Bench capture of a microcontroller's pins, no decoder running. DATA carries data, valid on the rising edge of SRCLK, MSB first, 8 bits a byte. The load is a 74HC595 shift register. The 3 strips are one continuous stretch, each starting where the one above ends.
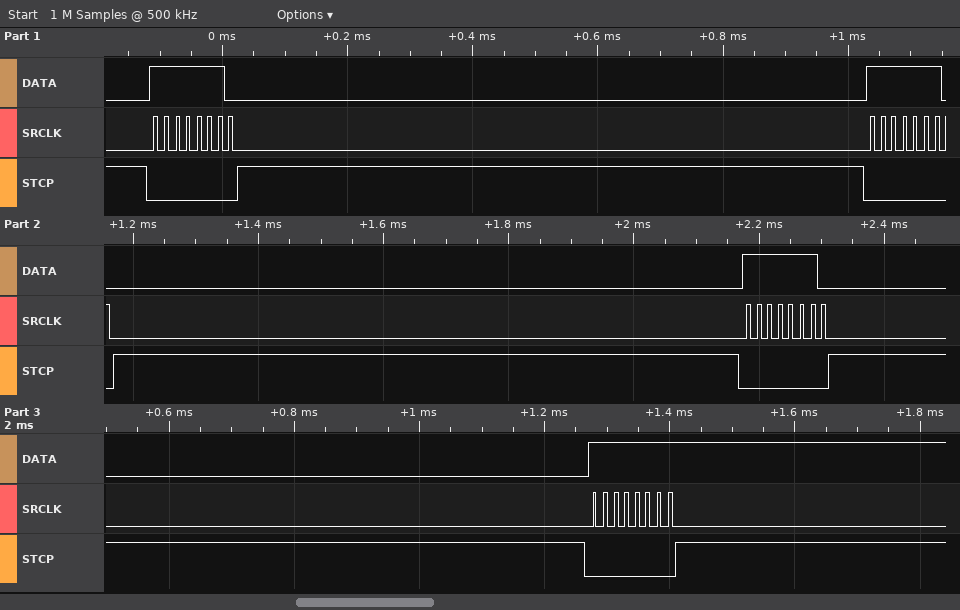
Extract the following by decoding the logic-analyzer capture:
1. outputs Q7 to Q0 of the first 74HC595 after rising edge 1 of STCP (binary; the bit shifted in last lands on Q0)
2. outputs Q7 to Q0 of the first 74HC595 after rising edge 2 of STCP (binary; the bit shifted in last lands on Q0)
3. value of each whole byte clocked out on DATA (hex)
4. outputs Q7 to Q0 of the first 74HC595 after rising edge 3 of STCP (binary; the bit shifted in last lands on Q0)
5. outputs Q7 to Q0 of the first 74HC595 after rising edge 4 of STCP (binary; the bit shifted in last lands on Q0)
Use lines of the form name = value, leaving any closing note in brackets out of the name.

outputs Q7 to Q0 of the first 74HC595 after rising edge 1 of STCP = 11111110
outputs Q7 to Q0 of the first 74HC595 after rising edge 2 of STCP = 11111110
value of each whole byte clocked out on DATA = 0xFE 0xFE 0xFE 0xFF
outputs Q7 to Q0 of the first 74HC595 after rising edge 3 of STCP = 11111110
outputs Q7 to Q0 of the first 74HC595 after rising edge 4 of STCP = 11111111
